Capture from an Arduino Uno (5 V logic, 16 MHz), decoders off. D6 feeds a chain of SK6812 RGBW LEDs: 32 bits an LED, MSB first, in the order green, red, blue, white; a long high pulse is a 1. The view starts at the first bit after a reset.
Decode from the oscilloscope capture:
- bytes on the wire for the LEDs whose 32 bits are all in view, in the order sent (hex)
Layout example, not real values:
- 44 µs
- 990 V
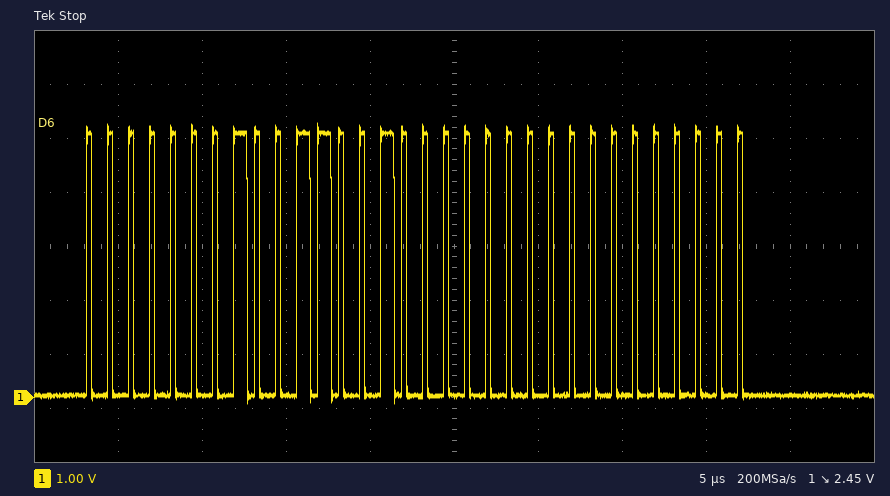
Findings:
- 01 32 00 00
